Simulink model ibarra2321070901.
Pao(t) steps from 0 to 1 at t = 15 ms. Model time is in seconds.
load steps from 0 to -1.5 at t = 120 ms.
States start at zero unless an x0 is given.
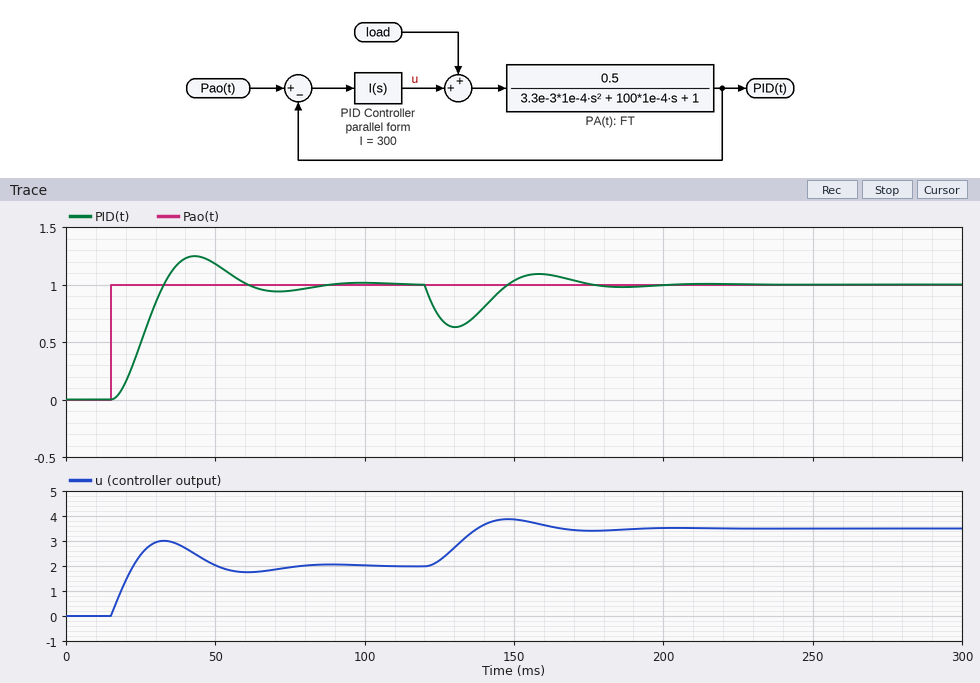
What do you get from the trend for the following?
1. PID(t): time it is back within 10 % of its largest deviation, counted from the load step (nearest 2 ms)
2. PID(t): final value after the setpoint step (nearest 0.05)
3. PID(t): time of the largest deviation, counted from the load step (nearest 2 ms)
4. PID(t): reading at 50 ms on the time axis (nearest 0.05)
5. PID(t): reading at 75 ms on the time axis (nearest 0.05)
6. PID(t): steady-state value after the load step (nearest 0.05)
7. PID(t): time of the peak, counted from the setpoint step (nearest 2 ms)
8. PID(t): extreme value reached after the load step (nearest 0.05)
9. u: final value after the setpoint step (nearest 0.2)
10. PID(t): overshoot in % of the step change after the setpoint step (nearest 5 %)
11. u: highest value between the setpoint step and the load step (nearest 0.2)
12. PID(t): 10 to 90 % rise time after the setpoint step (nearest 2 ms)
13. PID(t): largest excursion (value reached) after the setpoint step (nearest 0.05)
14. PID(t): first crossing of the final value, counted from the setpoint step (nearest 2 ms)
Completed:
50 ms
1.00
10 ms
1.20
0.95
1.00
28 ms
0.65
2.0
25 %
3.0
12 ms
1.25
18 ms
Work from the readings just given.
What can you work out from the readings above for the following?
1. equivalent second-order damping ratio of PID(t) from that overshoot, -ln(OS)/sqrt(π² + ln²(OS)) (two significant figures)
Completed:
0.40
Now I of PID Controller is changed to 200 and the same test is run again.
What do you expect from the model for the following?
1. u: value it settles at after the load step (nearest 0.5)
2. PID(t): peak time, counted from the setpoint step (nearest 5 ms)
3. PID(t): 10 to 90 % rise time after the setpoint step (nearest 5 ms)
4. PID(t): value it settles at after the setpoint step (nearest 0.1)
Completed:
3.5
35 ms
15 ms
1.0
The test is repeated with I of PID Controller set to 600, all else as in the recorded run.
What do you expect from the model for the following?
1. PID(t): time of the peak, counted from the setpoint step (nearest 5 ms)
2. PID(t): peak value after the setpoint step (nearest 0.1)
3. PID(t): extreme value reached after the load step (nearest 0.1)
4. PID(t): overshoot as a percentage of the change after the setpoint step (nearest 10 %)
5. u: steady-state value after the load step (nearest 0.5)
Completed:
20 ms
1.4
0.7
40 %
3.5
